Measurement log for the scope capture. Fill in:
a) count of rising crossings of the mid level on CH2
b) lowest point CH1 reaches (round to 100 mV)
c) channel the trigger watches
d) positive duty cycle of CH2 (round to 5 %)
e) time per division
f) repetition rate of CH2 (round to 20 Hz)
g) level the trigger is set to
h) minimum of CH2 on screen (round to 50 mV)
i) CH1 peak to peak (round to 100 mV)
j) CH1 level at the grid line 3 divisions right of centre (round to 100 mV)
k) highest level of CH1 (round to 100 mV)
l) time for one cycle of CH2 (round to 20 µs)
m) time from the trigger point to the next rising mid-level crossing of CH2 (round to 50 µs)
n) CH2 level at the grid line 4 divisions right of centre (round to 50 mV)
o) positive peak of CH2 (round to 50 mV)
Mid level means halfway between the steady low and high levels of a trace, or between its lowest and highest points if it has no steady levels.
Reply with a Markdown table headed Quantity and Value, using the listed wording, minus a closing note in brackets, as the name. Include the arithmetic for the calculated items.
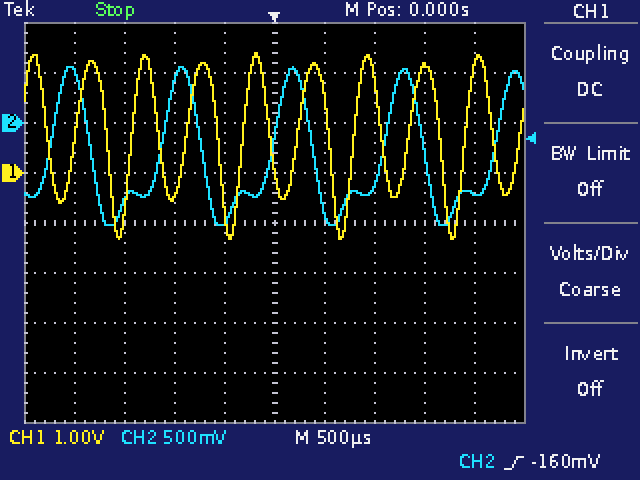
| Quantity | Value |
|---|---|
| count of rising crossings of the mid level on CH2 | 5 |
| lowest point CH1 reaches | -1.3 V |
| channel the trigger watches | CH2 |
| positive duty cycle of CH2 | 35 % |
| time per division | 500 µs |
| repetition rate of CH2 | 1 / 1.12 ms ≈ 893 Hz, so 900 Hz to the nearest 20 Hz |
| level the trigger is set to | -160 mV |
| minimum of CH2 on screen | -1.00 V |
| CH1 peak to peak | 2.4 V − (-1.3 V) = 3.7 V |
| CH1 level at the grid line 3 divisions right of centre | 2.1 V |
| highest level of CH1 | 2.4 V |
| time for one cycle of CH2 | 1.12 ms |
| time from the trigger point to the next rising mid-level crossing of CH2 | 1.10 ms |
| CH2 level at the grid line 4 divisions right of centre | -700 mV |
| positive peak of CH2 | 550 mV |
